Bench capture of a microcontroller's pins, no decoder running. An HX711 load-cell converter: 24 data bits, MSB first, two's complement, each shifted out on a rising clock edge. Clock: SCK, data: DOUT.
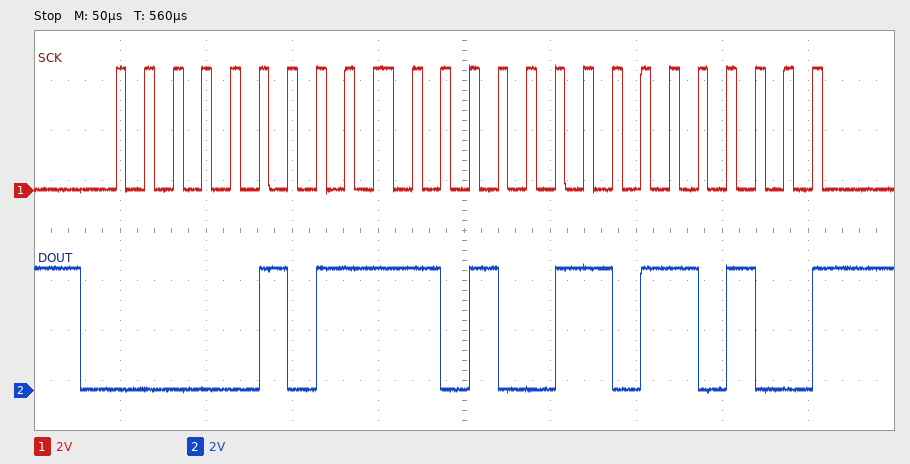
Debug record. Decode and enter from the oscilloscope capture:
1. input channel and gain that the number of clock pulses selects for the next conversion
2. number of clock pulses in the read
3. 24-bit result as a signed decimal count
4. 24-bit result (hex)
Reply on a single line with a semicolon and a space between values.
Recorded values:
channel A, gain 128; 25; 387508; 0x05E9B4
